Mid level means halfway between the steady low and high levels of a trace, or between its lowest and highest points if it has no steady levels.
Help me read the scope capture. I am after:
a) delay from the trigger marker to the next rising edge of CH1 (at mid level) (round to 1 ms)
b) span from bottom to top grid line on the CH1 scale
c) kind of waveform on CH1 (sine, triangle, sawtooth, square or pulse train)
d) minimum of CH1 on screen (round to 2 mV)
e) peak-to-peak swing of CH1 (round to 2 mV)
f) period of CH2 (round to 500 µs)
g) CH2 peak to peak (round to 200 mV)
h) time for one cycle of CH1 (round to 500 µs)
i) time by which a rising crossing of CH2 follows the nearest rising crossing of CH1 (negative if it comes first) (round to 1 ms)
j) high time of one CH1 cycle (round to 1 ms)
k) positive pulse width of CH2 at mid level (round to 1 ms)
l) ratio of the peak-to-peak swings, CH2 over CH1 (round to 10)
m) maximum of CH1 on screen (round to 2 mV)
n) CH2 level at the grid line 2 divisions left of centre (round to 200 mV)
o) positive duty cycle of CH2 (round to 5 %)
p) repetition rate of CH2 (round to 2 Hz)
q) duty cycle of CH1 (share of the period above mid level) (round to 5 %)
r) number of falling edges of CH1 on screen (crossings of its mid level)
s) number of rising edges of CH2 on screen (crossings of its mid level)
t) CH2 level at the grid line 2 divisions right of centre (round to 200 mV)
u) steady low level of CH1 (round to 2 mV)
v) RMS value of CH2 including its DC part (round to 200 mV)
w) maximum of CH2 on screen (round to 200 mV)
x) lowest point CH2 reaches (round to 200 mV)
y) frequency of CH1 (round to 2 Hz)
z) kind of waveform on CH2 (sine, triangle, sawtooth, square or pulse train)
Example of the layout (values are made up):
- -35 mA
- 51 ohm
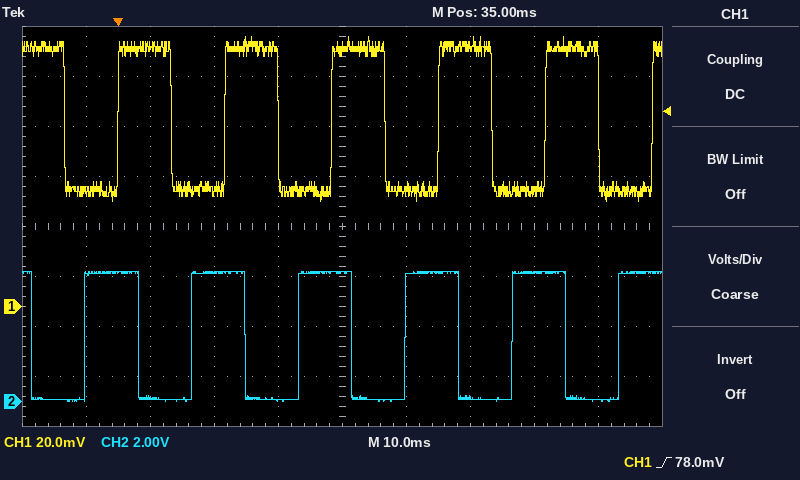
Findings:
- 17 ms
- 160 mV
- square
- 42 mV
- 66 mV
- 16.5 ms
- 5.2 V
- 16.5 ms
- -5 ms
- 8 ms
- 8 ms
- 80
- 108 mV
- 5.2 V
- 50 %
- 60 Hz
- 50 %
- 6
- 6
- 200 mV
- 46 mV
- 3.6 V
- 5.2 V
- 0.0 V
- 60 Hz
- square
